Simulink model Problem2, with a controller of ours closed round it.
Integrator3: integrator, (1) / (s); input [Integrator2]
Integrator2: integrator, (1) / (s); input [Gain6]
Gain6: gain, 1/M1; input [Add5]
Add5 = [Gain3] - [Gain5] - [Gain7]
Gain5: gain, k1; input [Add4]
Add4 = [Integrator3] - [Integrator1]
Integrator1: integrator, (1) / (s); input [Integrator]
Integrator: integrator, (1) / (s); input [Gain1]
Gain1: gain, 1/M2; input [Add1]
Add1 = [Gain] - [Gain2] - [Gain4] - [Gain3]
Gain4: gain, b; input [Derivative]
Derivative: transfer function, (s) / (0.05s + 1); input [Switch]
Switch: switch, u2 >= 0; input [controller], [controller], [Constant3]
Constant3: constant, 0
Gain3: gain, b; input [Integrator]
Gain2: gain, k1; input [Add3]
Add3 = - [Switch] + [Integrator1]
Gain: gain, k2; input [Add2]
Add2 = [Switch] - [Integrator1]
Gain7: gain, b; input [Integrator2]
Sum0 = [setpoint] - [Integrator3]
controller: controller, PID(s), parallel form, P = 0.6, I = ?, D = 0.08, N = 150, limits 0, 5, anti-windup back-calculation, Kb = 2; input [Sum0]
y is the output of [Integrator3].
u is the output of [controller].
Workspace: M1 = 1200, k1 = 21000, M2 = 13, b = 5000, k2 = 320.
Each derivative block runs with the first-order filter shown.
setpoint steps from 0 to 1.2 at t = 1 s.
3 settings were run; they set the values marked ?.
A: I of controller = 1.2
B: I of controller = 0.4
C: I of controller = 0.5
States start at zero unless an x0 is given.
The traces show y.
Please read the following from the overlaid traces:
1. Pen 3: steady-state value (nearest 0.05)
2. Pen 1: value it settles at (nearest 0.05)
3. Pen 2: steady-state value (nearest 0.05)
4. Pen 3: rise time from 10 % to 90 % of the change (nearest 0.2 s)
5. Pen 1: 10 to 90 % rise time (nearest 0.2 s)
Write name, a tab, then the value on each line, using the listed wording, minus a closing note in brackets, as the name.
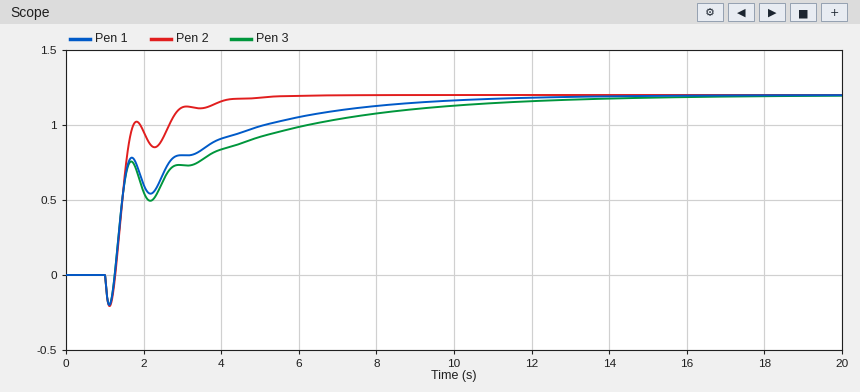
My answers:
Pen 3: steady-state value	1.20
Pen 1: value it settles at	1.20
Pen 2: steady-state value	1.20
Pen 3: rise time from 10 % to 90 % of the change	6.8 s
Pen 1: 10 to 90 % rise time	5.2 s
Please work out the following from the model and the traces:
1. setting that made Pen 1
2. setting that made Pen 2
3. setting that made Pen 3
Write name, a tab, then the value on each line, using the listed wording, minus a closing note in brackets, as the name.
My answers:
setting that made Pen 1	C
setting that made Pen 2	A
setting that made Pen 3	B
